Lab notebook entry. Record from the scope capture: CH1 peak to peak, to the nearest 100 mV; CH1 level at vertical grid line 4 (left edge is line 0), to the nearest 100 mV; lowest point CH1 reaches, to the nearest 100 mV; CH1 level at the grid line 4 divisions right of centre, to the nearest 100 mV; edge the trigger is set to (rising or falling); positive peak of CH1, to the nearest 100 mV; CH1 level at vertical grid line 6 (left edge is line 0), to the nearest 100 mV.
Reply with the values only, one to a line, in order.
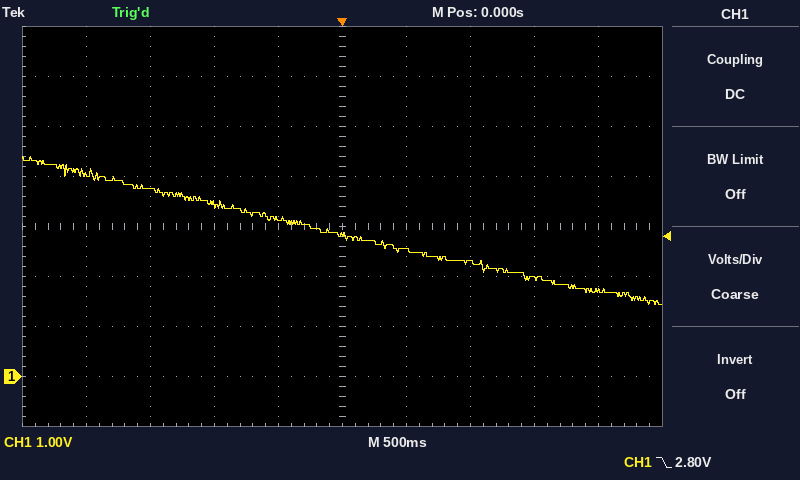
3.0 V
3.2 V
1.4 V
1.7 V
falling
4.4 V
2.5 V
